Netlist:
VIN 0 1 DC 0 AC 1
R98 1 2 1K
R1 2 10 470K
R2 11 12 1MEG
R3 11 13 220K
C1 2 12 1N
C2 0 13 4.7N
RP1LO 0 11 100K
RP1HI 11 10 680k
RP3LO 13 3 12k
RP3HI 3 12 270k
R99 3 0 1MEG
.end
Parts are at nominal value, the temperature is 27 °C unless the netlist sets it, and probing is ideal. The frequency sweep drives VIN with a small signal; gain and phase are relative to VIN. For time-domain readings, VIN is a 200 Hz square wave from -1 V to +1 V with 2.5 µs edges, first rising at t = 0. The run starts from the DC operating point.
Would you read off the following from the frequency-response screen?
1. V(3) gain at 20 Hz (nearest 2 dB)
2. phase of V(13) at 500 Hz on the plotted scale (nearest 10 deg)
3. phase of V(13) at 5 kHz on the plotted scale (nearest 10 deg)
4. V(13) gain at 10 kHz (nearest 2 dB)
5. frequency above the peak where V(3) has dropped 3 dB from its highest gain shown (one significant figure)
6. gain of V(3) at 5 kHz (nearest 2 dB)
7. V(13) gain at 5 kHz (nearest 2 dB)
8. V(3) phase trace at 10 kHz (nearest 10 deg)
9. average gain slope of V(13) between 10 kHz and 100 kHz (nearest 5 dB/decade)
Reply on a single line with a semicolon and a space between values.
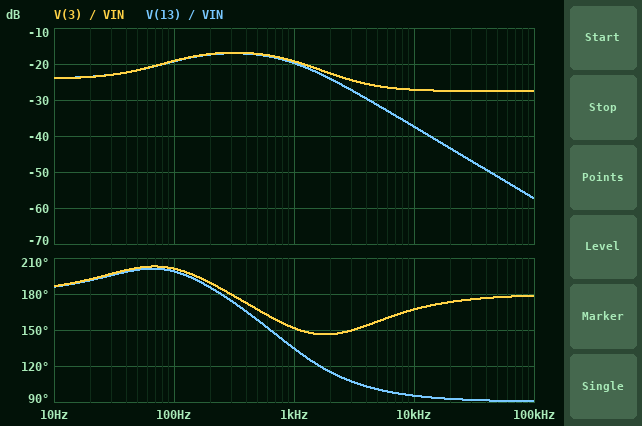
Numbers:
-24 dB; 160 deg; 100 deg; -38 dB; 1 kHz; -26 dB; -32 dB; 170 deg; -20 dB/decade
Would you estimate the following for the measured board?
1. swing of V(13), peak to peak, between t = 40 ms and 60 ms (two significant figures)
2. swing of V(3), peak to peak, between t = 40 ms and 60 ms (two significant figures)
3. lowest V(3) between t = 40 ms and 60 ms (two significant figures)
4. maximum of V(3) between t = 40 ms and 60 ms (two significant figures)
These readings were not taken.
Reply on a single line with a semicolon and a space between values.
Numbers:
350 mV; 360 mV; -180 mV; 180 mV
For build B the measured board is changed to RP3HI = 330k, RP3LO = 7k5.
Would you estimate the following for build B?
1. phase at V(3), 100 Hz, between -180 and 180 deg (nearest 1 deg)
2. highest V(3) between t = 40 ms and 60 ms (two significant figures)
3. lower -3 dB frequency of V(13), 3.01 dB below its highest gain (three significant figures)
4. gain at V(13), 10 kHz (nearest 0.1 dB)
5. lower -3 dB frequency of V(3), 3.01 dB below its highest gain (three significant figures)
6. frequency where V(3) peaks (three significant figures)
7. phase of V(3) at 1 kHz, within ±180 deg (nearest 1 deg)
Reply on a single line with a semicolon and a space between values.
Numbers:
-161 deg; 170 mV; 77.3 Hz; -38.7 dB; 78.3 Hz; 294 Hz; 141 deg
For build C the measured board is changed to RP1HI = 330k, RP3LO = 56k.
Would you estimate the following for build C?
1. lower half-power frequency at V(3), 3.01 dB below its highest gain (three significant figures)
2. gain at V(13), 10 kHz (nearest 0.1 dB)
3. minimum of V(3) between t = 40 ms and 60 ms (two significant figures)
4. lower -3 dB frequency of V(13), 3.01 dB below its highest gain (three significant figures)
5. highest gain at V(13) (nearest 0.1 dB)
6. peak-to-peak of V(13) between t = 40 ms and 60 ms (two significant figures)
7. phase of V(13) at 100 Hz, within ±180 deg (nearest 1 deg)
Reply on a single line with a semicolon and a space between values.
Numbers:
86.1 Hz; -38.5 dB; -220 mV; 47.1 Hz; -17.1 dB; 320 mV; -171 deg
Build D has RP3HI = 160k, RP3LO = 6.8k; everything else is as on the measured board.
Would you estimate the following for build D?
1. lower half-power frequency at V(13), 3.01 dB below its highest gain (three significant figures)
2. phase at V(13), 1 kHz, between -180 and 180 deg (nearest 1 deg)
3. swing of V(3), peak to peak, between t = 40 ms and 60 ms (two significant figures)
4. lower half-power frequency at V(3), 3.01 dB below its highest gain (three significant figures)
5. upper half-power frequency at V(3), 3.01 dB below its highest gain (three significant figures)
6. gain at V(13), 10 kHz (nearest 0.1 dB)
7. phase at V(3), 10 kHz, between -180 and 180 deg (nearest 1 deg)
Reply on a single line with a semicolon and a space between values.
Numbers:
90.5 Hz; 147 deg; 400 mV; 91.6 Hz; 1.64 kHz; -33.3 dB; 159 deg
